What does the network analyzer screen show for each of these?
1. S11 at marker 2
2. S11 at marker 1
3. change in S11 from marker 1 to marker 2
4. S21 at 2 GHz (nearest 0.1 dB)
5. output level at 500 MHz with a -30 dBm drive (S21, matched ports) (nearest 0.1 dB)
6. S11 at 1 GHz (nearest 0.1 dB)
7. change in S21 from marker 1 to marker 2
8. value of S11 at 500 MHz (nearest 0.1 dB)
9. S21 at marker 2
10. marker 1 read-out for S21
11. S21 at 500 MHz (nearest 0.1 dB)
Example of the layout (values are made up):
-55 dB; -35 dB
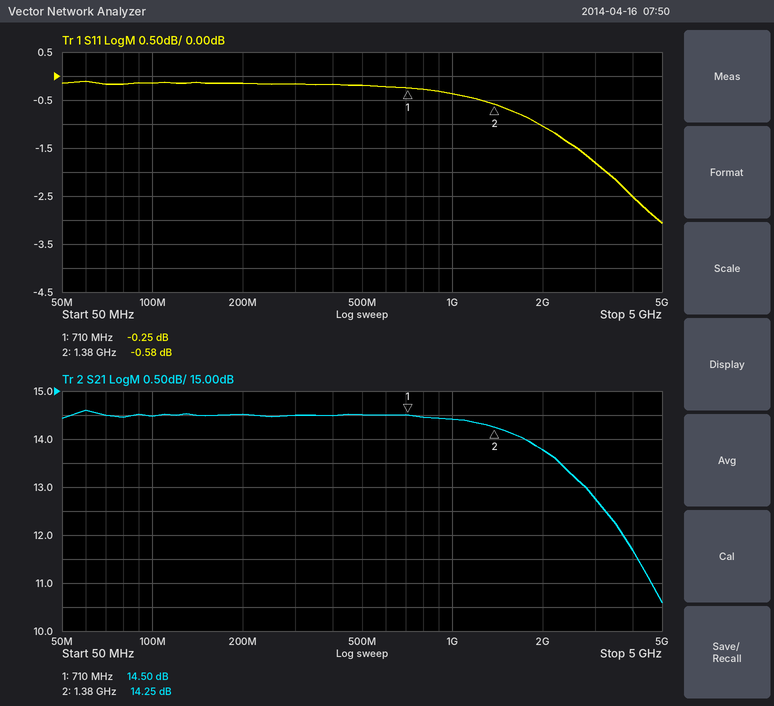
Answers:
-0.58 dB; -0.25 dB; -0.33 dB; 13.8 dB; -15.5 dBm; -0.4 dB; -0.25 dB; -0.2 dB; 14.25 dB; 14.50 dB; 14.5 dB
